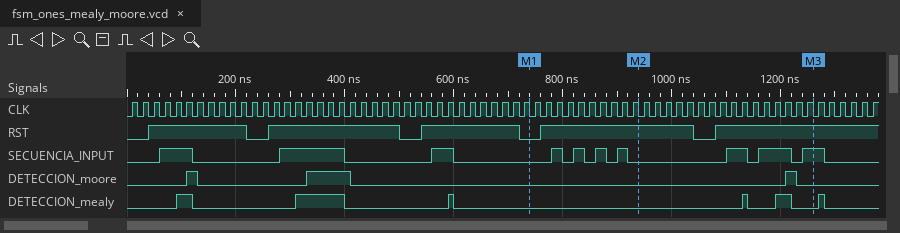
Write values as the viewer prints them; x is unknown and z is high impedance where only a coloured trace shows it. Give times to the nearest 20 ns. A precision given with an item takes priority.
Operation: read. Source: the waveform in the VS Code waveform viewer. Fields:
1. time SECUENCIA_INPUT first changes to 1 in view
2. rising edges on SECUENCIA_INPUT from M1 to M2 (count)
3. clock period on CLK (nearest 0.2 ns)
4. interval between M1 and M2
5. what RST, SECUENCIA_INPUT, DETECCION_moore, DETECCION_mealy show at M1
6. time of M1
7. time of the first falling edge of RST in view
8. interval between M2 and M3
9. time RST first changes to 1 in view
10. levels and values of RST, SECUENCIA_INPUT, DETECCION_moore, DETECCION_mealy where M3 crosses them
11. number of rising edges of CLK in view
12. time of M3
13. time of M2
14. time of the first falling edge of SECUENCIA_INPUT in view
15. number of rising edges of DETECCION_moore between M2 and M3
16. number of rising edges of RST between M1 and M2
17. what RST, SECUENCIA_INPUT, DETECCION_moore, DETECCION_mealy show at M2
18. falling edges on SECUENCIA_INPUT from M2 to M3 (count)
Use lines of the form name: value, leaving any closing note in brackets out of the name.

time SECUENCIA_INPUT first changes to 1 in view: 60 ns
rising edges on SECUENCIA_INPUT from M1 to M2: 4
clock period on CLK: 20 ns
interval between M1 and M2: 200 ns
what RST, SECUENCIA_INPUT, DETECCION_moore, DETECCION_mealy show at M1: RST=0, SECUENCIA_INPUT=0, DETECCION_moore=0, DETECCION_mealy=0
time of M1: 740 ns
time of the first falling edge of RST in view: 220 ns
interval between M2 and M3: 320 ns
time RST first changes to 1 in view: 40 ns
levels and values of RST, SECUENCIA_INPUT, DETECCION_moore, DETECCION_mealy where M3 crosses them: RST=1, SECUENCIA_INPUT=1, DETECCION_moore=0, DETECCION_mealy=0
number of rising edges of CLK in view: 69
time of M3: 1260 ns
time of M2: 940 ns
time of the first falling edge of SECUENCIA_INPUT in view: 120 ns
number of rising edges of DETECCION_moore between M2 and M3: 1
number of rising edges of RST between M1 and M2: 1
what RST, SECUENCIA_INPUT, DETECCION_moore, DETECCION_mealy show at M2: RST=1, SECUENCIA_INPUT=0, DETECCION_moore=0, DETECCION_mealy=0
falling edges on SECUENCIA_INPUT from M2 to M3: 2
